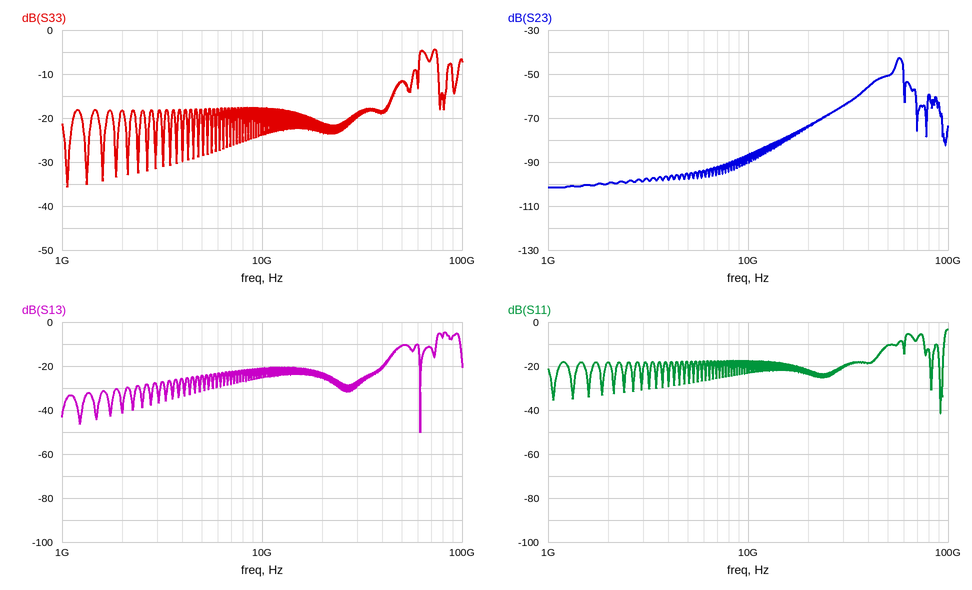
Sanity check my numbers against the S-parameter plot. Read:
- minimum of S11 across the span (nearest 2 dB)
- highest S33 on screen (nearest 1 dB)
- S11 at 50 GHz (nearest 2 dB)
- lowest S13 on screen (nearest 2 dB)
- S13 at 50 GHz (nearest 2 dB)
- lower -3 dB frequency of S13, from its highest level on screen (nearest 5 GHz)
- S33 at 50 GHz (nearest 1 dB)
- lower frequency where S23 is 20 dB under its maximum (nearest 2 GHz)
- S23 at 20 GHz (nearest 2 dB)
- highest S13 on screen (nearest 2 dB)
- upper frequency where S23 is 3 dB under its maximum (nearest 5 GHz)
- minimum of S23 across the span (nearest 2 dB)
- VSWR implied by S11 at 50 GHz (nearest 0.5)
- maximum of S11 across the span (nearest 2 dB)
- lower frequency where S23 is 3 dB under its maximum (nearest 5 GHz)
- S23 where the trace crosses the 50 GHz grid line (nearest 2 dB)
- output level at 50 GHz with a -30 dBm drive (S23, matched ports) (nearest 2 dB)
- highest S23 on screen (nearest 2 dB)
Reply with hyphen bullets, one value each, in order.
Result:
- -42 dB
- -4 dB
- -10 dB
- -50 dB
- -10 dB
- 75 GHz
- -12 dB
- 32 GHz
- -74 dB
- -4 dB
- 60 GHz
- -102 dB
- 2.0
- -4 dB
- 55 GHz
- -50 dB
- -80 dBm
- -42 dB
